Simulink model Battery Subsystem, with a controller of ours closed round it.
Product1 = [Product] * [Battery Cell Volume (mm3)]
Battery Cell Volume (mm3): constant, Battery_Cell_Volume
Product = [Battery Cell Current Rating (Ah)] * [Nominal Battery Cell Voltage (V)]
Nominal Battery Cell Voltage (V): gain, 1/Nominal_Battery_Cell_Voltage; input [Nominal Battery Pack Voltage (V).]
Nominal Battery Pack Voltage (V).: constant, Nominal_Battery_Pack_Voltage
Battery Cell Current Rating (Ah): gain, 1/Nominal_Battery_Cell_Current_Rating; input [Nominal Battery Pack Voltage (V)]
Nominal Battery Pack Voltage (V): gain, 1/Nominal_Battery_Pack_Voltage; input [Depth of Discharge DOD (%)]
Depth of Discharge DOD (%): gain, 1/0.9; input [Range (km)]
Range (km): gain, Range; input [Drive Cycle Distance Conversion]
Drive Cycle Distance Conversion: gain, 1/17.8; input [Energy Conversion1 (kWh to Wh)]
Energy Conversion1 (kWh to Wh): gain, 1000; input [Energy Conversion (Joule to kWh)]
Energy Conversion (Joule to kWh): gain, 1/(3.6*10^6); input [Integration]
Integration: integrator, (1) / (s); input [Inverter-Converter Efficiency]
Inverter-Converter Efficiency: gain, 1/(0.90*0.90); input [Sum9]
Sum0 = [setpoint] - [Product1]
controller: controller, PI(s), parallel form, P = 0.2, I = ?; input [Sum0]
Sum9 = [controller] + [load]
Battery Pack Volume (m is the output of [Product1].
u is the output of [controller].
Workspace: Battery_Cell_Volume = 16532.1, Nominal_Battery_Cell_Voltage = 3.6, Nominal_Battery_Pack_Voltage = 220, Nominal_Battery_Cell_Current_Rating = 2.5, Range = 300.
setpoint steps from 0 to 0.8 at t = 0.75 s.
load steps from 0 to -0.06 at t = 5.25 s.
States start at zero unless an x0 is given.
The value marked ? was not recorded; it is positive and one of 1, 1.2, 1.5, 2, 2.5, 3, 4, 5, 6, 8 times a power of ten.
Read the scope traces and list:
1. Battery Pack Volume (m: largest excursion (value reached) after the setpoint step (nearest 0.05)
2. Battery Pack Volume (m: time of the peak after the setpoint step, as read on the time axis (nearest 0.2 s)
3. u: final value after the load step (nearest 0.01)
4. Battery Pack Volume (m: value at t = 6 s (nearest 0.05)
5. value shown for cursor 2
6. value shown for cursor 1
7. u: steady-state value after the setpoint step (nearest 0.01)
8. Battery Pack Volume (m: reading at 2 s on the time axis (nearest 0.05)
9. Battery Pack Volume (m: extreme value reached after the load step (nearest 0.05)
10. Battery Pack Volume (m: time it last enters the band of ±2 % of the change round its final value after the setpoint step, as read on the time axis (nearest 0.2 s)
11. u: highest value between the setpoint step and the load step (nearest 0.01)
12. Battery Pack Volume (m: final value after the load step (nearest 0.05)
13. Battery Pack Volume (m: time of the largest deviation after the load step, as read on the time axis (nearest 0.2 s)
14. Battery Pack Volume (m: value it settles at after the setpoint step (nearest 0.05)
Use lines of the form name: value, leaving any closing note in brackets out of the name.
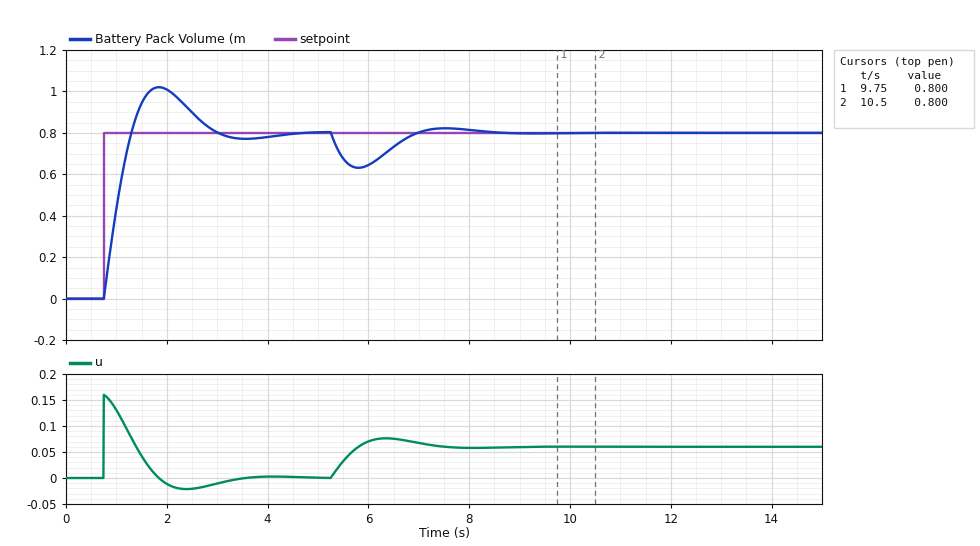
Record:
Battery Pack Volume (m: largest excursion (value reached) after the setpoint step: 1.00
Battery Pack Volume (m: time of the peak after the setpoint step, as read on the time axis: 1.8 s
u: final value after the load step: 0.06
Battery Pack Volume (m: value at t = 6 s: 0.65
value shown for cursor 2: 0.800
value shown for cursor 1: 0.800
u: steady-state value after the setpoint step: 0.00
Battery Pack Volume (m: reading at 2 s on the time axis: 1.00
Battery Pack Volume (m: extreme value reached after the load step: 0.65
Battery Pack Volume (m: time it last enters the band of ±2 % of the change round its final value after the setpoint step, as read on the time axis: 4.2 s
u: highest value between the setpoint step and the load step: 0.16
Battery Pack Volume (m: final value after the load step: 0.80
Battery Pack Volume (m: time of the largest deviation after the load step, as read on the time axis: 5.8 s
Battery Pack Volume (m: value it settles at after the setpoint step: 0.80
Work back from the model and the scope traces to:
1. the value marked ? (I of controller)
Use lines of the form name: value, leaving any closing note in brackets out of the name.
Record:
the value marked ?: 0.4
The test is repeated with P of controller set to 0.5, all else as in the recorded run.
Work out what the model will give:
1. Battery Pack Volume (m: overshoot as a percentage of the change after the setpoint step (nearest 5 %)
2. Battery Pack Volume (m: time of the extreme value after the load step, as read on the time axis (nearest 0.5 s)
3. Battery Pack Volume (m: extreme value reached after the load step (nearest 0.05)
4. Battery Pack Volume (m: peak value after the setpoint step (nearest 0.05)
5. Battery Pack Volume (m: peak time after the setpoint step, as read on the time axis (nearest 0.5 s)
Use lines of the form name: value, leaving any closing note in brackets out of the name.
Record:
Battery Pack Volume (m: overshoot as a percentage of the change after the setpoint step: 10 %
Battery Pack Volume (m: time of the extreme value after the load step, as read on the time axis: 5.5 s
Battery Pack Volume (m: extreme value reached after the load step: 0.70
Battery Pack Volume (m: peak value after the setpoint step: 0.85
Battery Pack Volume (m: peak time after the setpoint step, as read on the time axis: 1.5 s
